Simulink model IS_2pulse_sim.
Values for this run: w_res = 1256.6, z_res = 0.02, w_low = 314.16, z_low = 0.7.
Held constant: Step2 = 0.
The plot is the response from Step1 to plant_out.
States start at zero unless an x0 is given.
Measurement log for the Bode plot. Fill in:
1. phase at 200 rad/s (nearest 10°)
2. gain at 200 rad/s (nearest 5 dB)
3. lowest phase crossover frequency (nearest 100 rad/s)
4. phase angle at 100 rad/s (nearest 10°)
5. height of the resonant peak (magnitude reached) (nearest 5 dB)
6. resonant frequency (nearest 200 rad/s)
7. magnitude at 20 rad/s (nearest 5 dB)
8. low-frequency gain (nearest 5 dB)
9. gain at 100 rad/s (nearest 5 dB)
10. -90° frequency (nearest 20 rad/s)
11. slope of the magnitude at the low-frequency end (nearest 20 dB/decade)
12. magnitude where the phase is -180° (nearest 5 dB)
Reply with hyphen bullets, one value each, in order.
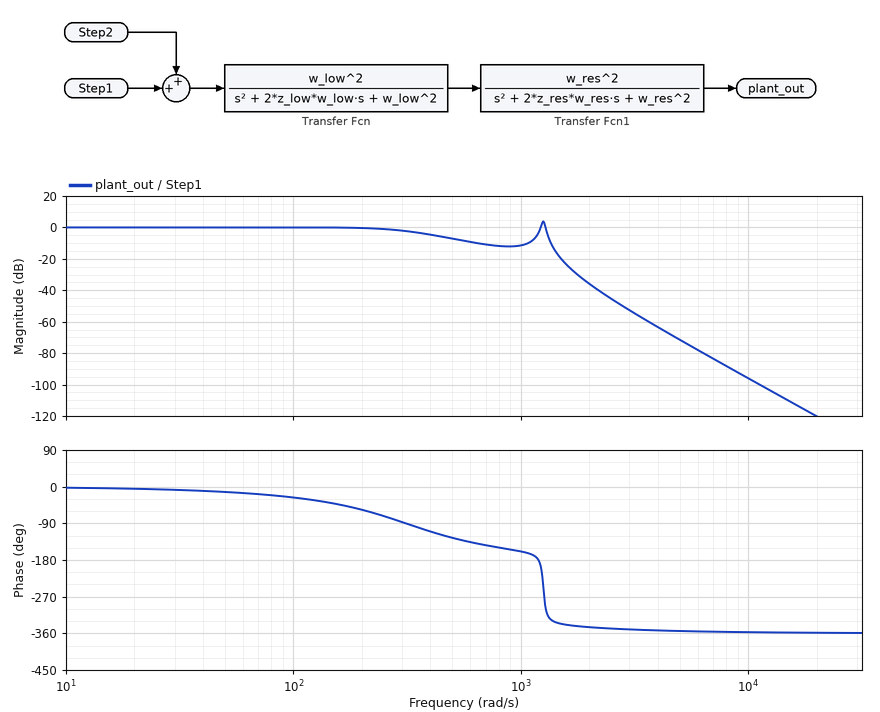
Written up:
- -60°
- 0 dB
- 1200 rad/s
- -30°
- 5 dB
- 1200 rad/s
- 0 dB
- 0 dB
- 0 dB
- 320 rad/s
- 0 dB/decade
- -5 dB
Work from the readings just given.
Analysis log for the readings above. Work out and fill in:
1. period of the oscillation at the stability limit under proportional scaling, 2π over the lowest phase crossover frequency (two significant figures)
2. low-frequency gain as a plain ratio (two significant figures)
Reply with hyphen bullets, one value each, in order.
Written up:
- 0.0052 s
- 1.0
